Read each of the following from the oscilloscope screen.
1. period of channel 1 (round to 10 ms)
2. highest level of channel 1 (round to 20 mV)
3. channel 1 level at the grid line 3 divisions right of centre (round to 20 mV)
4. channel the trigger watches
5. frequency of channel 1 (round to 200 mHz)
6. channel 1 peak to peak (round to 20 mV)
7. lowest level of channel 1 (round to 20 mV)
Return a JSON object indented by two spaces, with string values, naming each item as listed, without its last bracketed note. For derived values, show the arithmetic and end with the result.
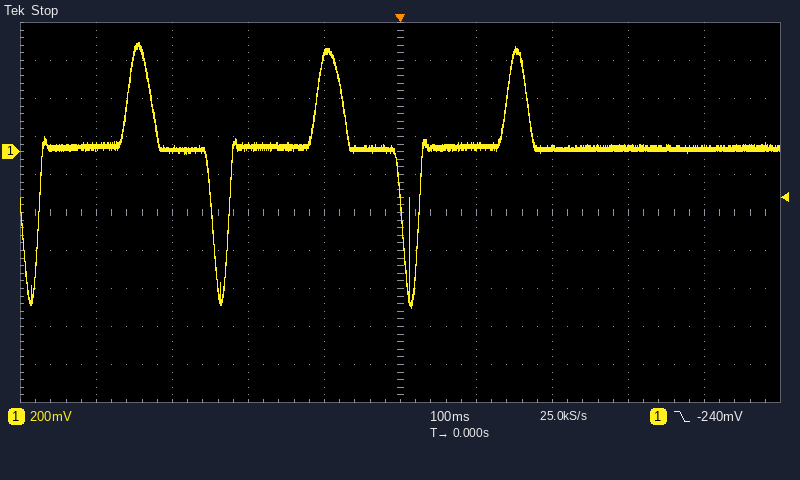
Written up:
{
  "period of channel 1": "250 ms",
  "highest level of channel 1": "580 mV",
  "channel 1 level at the grid line 3 divisions right of centre": "20 mV",
  "channel the trigger watches": "channel 1",
  "frequency of channel 1": "1 / 250 ms ≈ 4.0 Hz",
  "channel 1 peak to peak": "580 mV − (-820 mV) = 1.40 V",
  "lowest level of channel 1": "-820 mV"
}
